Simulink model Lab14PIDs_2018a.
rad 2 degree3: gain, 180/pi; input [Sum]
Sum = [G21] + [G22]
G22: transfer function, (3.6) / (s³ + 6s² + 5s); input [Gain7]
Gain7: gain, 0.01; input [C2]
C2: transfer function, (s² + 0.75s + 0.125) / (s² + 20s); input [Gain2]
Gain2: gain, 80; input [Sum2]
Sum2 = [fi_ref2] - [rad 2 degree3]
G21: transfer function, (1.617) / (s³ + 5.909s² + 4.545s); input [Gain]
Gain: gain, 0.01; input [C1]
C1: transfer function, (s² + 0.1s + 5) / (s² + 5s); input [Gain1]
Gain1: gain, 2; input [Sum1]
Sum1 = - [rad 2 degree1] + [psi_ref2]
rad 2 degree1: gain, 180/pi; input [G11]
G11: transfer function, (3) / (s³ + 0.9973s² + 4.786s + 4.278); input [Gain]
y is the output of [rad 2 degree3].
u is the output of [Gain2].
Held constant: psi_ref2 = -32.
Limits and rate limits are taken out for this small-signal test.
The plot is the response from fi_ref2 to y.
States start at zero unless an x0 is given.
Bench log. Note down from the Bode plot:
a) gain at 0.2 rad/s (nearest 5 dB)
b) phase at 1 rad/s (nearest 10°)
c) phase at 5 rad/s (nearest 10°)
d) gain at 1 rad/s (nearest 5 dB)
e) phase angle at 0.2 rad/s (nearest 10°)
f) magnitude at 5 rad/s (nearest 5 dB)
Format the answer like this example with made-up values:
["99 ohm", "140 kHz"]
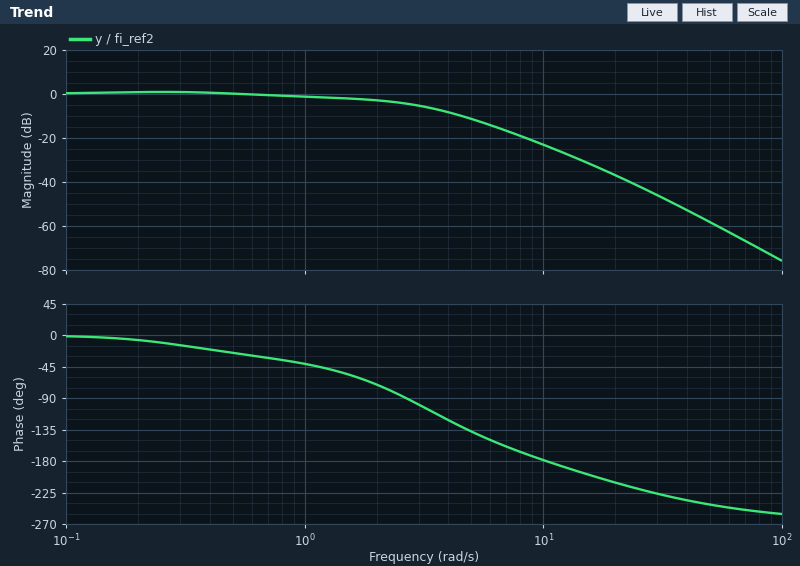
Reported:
["0 dB", "-40°", "-140°", "0 dB", "-10°", "-10 dB"]
